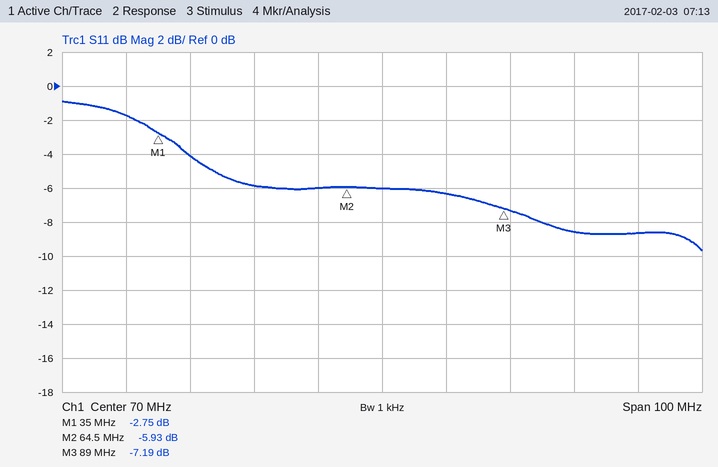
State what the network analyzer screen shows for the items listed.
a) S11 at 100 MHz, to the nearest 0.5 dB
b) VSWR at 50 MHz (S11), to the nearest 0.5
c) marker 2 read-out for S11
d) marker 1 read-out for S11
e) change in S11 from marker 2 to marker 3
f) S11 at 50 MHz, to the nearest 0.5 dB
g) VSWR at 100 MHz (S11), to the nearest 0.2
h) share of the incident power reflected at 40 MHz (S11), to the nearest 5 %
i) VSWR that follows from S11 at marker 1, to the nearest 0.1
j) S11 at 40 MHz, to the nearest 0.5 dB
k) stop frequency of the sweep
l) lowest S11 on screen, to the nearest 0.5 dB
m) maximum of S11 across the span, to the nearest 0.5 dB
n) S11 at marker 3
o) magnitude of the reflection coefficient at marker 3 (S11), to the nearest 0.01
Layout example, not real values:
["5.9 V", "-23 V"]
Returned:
["-8.5 dB", "3.0", "-5.93 dB", "-2.75 dB", "-1.26 dB", "-6.0 dB", "2.2", "40 %", "6.4", "-4.0 dB", "120 MHz", "-9.5 dB", "-1.0 dB", "-7.19 dB", "0.44"]
